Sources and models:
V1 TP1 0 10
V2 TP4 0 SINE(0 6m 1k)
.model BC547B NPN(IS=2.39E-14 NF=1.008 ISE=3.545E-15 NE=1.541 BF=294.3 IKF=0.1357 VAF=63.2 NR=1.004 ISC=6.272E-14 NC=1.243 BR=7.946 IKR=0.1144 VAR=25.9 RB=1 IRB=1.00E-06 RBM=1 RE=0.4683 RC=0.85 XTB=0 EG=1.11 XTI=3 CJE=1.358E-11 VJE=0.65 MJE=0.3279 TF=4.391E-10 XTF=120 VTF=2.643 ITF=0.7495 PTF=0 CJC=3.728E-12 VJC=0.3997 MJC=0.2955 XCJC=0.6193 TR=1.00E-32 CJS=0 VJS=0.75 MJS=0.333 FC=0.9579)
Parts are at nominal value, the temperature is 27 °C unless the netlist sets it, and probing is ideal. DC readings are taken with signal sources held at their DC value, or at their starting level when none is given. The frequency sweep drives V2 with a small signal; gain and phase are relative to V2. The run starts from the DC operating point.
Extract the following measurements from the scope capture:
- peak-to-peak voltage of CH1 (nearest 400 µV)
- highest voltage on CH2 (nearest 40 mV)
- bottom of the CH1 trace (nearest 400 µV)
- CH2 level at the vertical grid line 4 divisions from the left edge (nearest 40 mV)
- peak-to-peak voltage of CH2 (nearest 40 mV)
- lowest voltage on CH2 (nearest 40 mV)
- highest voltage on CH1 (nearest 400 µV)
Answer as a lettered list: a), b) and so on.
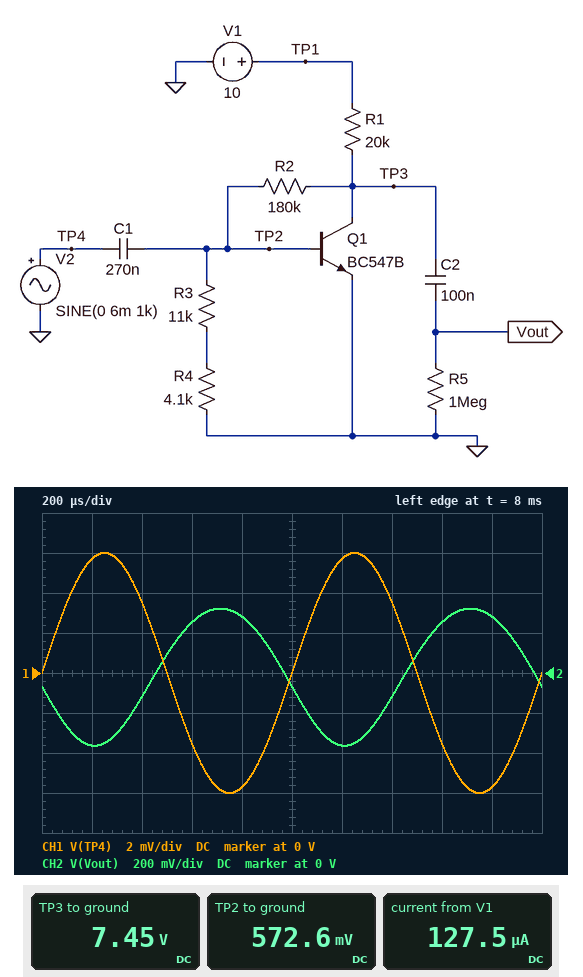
a) 12.0 mV
b) 320 mV
c) -6.0 mV
d) 280 mV
e) 680 mV
f) -360 mV
g) 6.0 mV
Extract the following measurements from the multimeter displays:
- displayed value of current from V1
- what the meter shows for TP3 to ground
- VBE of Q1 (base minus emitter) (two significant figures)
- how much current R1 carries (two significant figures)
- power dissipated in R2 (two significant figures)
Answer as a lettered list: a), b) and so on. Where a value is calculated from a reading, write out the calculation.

a) 127.5 µA
b) 7.45 V
c) 572.6 mV = 570 mV
d) (10 V - 7.45 V) / 20 kΩ = 130 µA
e) (7.45 V - 572.6 mV)^2 / 180 kΩ = 260 µW
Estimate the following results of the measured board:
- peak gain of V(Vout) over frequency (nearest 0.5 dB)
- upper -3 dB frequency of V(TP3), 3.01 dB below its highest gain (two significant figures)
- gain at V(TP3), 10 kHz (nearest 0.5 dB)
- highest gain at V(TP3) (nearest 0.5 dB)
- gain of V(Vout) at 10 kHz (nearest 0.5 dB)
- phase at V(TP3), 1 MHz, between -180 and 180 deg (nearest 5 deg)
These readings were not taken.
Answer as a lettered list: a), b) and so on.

a) 35.5 dB
b) 5.8 MHz
c) 35.5 dB
d) 35.5 dB
e) 35.5 dB
f) 170 deg
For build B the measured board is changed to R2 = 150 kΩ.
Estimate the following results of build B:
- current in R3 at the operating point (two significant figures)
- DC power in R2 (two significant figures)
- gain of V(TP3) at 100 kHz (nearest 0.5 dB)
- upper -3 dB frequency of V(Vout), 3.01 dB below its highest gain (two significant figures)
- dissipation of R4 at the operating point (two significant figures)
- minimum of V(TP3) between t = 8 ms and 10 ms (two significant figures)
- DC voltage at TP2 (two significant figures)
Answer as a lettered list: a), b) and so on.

a) 39 µA
b) 230 µW
c) 39.0 dB
d) 5.7 MHz
e) 6.1 µW
f) 5.9 V
g) 580 mV
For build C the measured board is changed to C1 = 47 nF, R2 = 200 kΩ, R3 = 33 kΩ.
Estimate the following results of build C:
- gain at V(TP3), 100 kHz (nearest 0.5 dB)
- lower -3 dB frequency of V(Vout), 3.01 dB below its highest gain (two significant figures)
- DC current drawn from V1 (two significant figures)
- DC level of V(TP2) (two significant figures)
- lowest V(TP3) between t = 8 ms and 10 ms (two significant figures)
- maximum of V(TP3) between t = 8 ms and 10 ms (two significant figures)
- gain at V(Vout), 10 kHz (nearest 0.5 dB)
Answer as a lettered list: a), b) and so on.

a) 45.0 dB
b) 3.2 kHz
c) 300 µA
d) 600 mV
e) 3.7 V
f) 4.4 V
g) 44.5 dB
